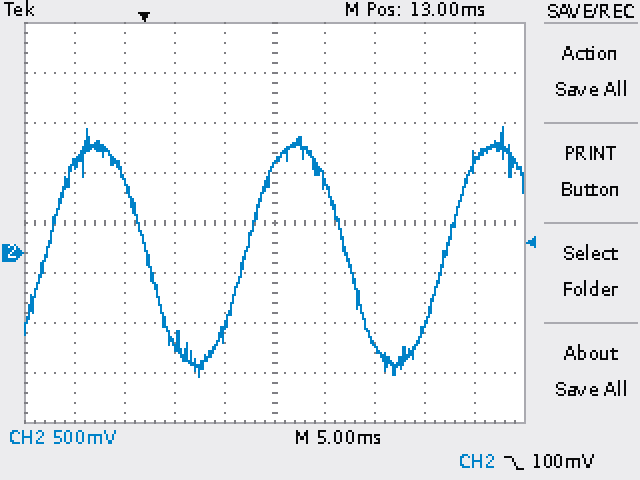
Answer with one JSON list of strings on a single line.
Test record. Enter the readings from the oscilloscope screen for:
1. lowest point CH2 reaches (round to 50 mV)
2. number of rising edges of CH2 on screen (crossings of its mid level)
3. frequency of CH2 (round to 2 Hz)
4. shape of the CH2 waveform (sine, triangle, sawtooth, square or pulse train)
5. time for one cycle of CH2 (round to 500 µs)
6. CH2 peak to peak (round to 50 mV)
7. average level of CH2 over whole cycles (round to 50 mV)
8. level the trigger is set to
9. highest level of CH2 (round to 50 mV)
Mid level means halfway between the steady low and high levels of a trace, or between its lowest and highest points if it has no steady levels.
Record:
["-1.25 V", "3", "50 Hz", "sine", "20.0 ms", "2.50 V", "0 mV", "100 mV", "1.25 V"]
